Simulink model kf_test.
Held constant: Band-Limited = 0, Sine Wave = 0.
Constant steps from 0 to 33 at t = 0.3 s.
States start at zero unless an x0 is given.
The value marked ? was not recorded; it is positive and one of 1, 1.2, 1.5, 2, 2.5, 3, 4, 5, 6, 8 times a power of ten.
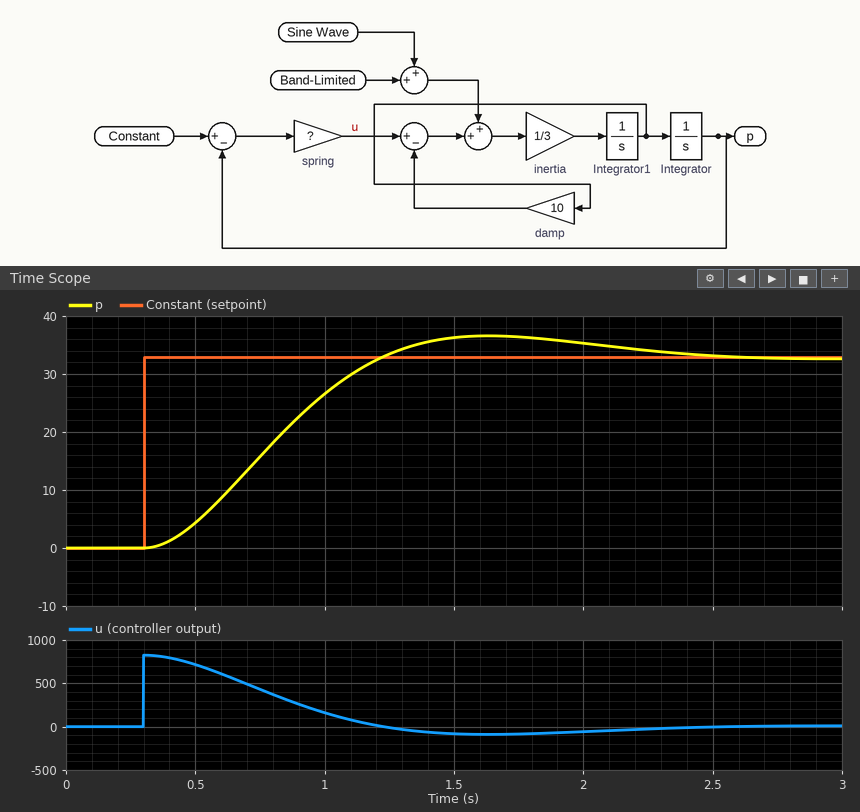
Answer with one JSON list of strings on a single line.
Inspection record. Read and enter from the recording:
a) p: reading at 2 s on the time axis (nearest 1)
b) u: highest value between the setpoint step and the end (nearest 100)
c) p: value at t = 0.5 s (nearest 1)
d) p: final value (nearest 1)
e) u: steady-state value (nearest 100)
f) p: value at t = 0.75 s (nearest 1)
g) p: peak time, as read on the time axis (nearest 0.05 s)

["35", "800", "4", "33", "0", "16", "1.65 s"]
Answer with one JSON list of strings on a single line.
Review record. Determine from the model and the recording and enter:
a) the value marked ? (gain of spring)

["25"]
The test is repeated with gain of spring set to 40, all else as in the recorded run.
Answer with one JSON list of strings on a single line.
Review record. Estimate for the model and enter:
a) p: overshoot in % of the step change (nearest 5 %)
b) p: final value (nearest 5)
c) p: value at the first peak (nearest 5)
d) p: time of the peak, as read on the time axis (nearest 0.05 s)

["20 %", "35", "40", "1.25 s"]
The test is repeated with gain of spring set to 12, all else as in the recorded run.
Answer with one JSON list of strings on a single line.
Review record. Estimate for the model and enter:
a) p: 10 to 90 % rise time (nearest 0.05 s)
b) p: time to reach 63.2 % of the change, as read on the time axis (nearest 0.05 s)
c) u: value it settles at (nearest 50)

["1.30 s", "1.25 s", "0"]
